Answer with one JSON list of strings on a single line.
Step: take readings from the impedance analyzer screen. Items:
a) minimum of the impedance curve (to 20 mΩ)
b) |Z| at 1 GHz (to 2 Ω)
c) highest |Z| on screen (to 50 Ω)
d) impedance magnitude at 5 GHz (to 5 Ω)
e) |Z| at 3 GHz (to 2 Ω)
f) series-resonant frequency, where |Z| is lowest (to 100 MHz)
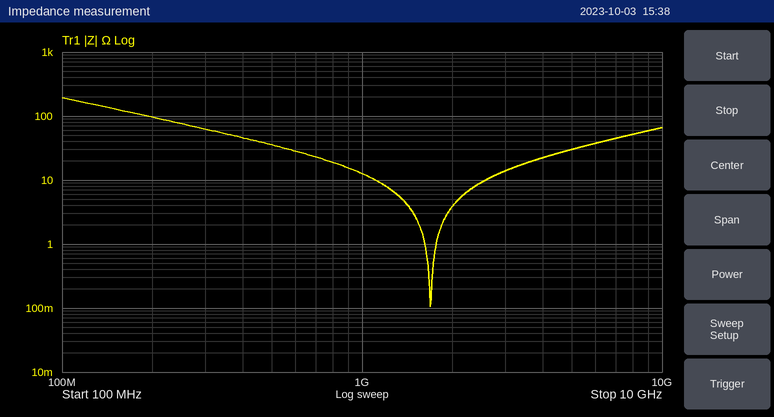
["100 mΩ", "12 Ω", "200 Ω", "30 Ω", "14 Ω", "1.7 GHz"]
